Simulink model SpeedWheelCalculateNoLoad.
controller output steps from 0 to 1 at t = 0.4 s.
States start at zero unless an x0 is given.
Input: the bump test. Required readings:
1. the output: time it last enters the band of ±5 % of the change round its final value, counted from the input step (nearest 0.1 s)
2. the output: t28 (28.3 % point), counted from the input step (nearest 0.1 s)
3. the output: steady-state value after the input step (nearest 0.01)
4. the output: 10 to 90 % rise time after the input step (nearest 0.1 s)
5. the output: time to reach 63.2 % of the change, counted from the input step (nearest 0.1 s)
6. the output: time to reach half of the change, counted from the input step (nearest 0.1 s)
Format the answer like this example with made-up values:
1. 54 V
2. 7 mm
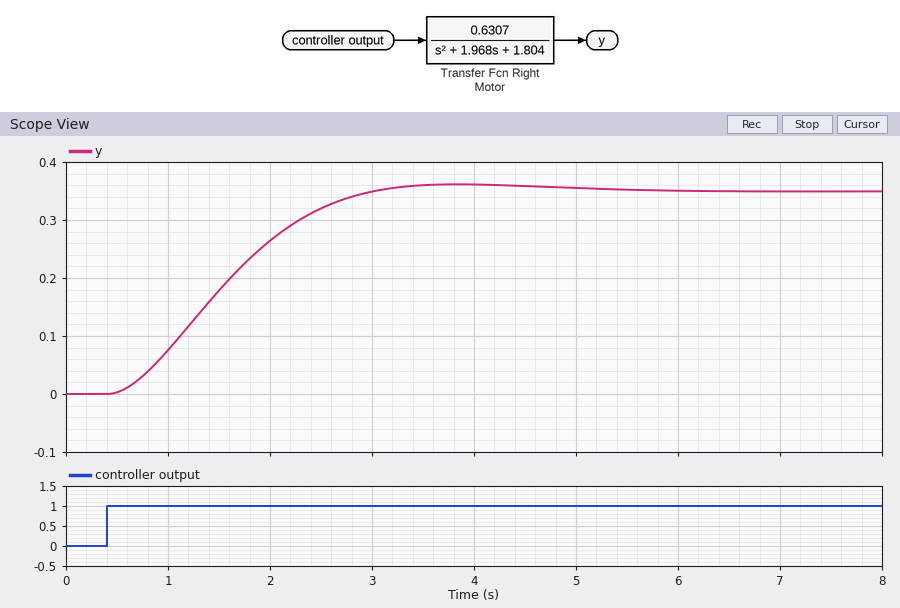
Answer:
1. 2.3 s
2. 0.7 s
3. 0.35
4. 1.7 s
5. 1.3 s
6. 1.1 s
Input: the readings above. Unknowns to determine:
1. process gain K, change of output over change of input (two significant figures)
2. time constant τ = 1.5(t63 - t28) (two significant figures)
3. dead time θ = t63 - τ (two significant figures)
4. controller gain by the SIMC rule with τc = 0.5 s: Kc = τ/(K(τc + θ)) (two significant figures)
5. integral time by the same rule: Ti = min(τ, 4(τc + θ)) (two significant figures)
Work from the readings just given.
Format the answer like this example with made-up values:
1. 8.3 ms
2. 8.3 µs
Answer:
1. 0.35
2. 0.90 s
3. 0.40 s
4. 2.9
5. 0.90 s
